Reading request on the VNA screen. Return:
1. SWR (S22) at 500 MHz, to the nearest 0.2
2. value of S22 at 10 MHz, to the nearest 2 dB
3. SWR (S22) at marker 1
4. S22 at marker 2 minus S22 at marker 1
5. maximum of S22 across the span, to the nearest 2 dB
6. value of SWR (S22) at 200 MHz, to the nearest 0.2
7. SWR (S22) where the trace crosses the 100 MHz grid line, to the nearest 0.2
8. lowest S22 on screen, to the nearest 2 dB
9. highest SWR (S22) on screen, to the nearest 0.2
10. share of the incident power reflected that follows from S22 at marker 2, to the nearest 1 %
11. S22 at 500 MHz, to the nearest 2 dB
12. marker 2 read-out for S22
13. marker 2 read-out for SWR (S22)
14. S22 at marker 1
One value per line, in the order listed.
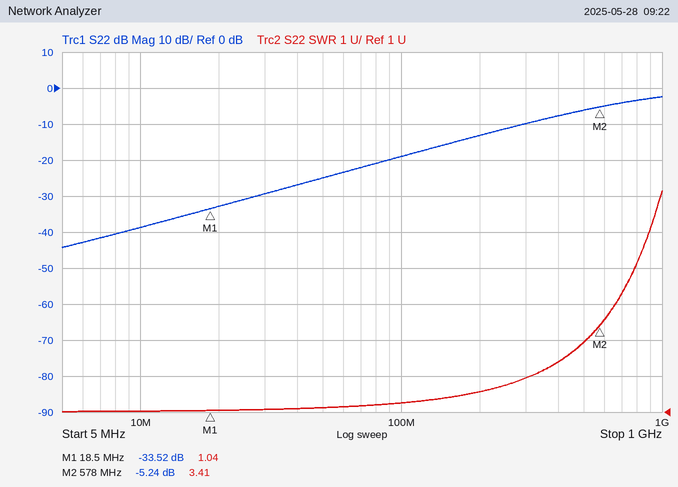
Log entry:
3.0
-38 dB
1.04
28.28 dB
-2 dB
1.6
1.2
-44 dB
7.2
30 %
-6 dB
-5.24 dB
3.41
-33.52 dB
